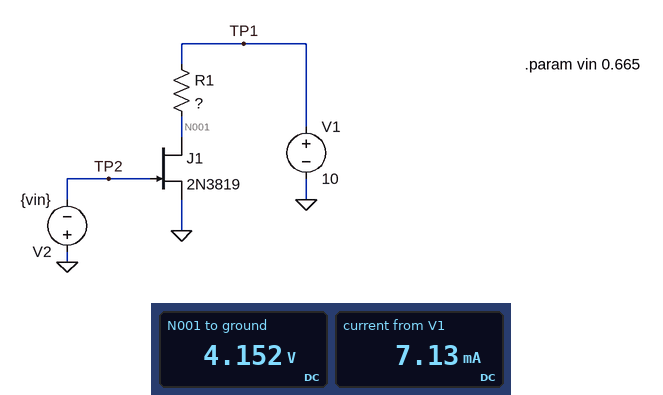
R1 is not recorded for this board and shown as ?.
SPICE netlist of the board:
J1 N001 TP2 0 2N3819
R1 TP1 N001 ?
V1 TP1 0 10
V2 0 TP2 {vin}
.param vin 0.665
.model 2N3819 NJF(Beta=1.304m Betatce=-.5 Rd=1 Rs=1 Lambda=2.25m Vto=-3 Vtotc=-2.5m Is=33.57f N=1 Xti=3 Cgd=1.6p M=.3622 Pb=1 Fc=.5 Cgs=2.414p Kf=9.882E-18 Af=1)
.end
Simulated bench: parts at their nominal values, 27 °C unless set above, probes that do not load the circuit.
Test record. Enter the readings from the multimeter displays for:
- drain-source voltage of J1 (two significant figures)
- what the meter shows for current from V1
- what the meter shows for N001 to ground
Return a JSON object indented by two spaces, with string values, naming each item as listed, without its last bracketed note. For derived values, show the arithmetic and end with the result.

{
  "drain-source voltage of J1": "4.152 V = 4.2 V",
  "what the meter shows for current from V1": "7.13 mA",
  "what the meter shows for N001 to ground": "4.152 V"
}
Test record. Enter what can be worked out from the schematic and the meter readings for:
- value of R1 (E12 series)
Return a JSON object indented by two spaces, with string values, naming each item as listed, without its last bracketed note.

{
  "value of R1": "820 Ω"
}
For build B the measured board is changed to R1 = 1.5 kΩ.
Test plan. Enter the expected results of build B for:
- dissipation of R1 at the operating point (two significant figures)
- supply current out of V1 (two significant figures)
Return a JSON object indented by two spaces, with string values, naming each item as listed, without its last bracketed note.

{
  "dissipation of R1 at the operating point": "50 mW",
  "supply current out of V1": "5.8 mA"
}
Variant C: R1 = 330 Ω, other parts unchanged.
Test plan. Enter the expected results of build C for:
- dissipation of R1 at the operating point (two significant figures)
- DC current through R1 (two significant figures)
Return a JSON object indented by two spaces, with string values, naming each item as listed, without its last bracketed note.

{
  "dissipation of R1 at the operating point": "17 mW",
  "DC current through R1": "7.2 mA"
}
